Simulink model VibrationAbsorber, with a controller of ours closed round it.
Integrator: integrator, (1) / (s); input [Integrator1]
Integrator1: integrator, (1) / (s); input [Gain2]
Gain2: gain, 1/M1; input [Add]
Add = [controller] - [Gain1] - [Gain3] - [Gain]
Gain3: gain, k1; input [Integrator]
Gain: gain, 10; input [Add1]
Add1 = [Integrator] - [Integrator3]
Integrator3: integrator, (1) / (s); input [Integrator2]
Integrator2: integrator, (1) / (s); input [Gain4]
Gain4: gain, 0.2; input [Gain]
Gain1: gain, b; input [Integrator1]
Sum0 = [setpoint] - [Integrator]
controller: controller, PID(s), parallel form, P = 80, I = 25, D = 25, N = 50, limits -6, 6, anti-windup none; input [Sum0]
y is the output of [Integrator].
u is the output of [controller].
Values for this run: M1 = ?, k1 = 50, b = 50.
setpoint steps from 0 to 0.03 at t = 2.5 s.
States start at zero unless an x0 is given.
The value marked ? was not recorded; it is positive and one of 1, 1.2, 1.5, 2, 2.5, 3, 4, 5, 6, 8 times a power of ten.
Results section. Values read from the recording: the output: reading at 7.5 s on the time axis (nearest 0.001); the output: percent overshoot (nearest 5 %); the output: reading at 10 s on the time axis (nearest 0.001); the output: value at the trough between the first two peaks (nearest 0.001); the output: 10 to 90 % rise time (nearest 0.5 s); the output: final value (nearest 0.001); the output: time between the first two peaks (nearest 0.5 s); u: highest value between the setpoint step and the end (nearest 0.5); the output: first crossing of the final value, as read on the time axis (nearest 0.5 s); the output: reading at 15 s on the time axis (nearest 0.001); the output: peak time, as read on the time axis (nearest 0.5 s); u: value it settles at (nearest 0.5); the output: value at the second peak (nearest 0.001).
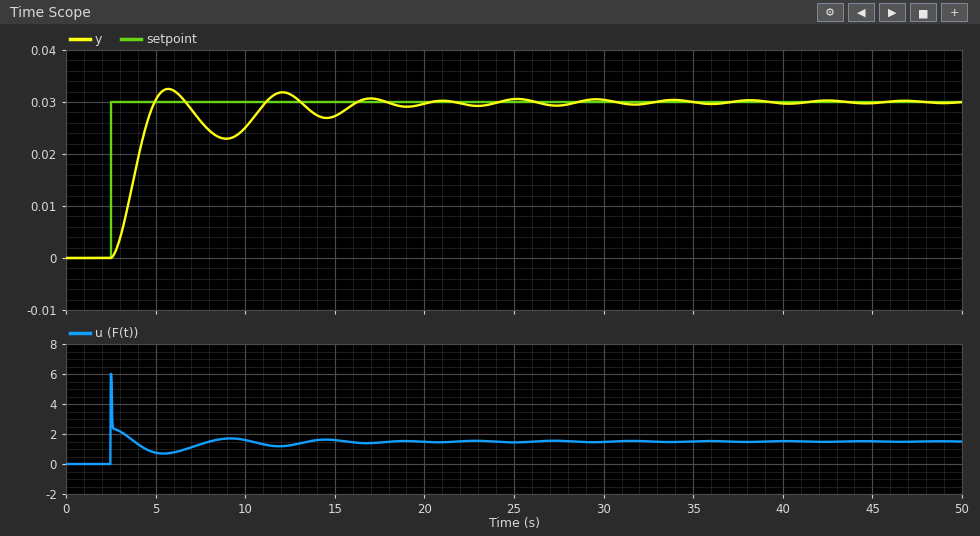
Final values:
0.026
10 %
0.025
0.023
1.5 s
0.030
6.5 s
6.0
5.0 s
0.027
5.5 s
1.5
0.032
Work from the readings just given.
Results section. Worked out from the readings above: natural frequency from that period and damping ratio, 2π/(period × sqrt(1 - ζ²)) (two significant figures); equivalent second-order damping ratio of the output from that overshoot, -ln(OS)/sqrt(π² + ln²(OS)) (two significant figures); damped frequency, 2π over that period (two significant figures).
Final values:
1.2 rad/s
0.59
0.97 rad/s
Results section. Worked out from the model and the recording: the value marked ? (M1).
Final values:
100
